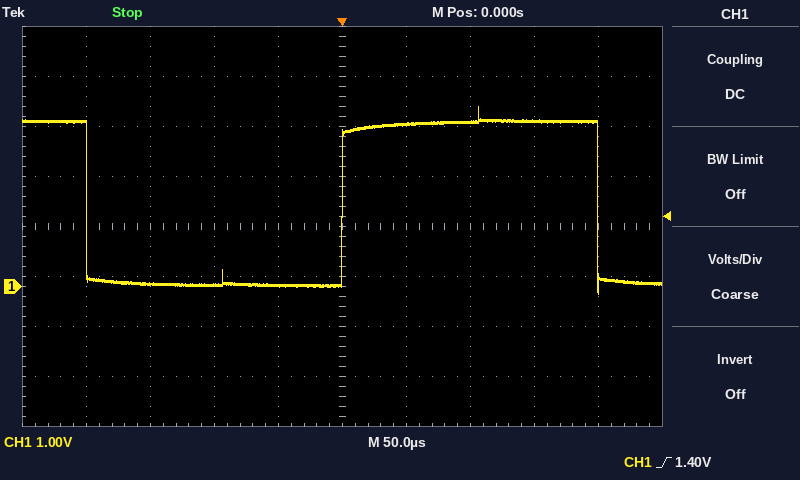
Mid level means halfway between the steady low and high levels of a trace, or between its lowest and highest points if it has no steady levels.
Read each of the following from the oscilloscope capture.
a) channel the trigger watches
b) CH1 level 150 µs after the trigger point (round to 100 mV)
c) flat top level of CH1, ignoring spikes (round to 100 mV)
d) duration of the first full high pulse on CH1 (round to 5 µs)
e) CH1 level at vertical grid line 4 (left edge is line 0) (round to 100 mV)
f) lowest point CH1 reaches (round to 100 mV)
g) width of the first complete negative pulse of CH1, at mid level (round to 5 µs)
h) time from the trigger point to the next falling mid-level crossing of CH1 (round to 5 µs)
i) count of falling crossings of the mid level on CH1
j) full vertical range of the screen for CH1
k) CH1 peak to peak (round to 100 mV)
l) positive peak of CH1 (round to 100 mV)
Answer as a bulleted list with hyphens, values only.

- CH1
- 3.3 V
- 3.3 V
- 200 µs
- 0.0 V
- -100 mV
- 200 µs
- 200 µs
- 2
- 8 V
- 3.7 V
- 3.6 V
